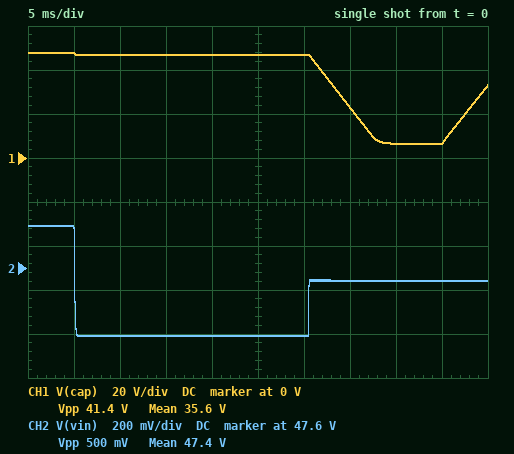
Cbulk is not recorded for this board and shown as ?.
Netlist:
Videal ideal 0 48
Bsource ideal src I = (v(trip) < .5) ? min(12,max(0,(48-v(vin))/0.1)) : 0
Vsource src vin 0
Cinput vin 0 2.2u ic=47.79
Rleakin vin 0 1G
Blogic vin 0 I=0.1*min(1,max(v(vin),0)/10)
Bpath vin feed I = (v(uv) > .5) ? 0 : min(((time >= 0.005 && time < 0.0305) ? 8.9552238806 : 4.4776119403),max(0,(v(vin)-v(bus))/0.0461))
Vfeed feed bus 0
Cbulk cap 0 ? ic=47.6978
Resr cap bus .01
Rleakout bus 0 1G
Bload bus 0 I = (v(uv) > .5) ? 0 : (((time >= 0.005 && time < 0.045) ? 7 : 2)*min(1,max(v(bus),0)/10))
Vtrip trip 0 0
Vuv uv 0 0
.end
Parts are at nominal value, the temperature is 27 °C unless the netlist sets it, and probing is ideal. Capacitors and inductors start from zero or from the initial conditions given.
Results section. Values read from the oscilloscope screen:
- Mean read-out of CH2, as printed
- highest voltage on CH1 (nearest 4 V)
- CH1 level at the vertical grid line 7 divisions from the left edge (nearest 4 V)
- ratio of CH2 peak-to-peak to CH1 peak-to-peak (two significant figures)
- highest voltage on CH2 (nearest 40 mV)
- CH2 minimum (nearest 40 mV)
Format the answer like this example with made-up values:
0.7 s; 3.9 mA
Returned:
47.4 V; 48 V; 24 V; 0.012; 47.80 V; 47.28 V
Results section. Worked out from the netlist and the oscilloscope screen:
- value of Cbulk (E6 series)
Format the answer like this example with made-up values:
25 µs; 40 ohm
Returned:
470 µF
